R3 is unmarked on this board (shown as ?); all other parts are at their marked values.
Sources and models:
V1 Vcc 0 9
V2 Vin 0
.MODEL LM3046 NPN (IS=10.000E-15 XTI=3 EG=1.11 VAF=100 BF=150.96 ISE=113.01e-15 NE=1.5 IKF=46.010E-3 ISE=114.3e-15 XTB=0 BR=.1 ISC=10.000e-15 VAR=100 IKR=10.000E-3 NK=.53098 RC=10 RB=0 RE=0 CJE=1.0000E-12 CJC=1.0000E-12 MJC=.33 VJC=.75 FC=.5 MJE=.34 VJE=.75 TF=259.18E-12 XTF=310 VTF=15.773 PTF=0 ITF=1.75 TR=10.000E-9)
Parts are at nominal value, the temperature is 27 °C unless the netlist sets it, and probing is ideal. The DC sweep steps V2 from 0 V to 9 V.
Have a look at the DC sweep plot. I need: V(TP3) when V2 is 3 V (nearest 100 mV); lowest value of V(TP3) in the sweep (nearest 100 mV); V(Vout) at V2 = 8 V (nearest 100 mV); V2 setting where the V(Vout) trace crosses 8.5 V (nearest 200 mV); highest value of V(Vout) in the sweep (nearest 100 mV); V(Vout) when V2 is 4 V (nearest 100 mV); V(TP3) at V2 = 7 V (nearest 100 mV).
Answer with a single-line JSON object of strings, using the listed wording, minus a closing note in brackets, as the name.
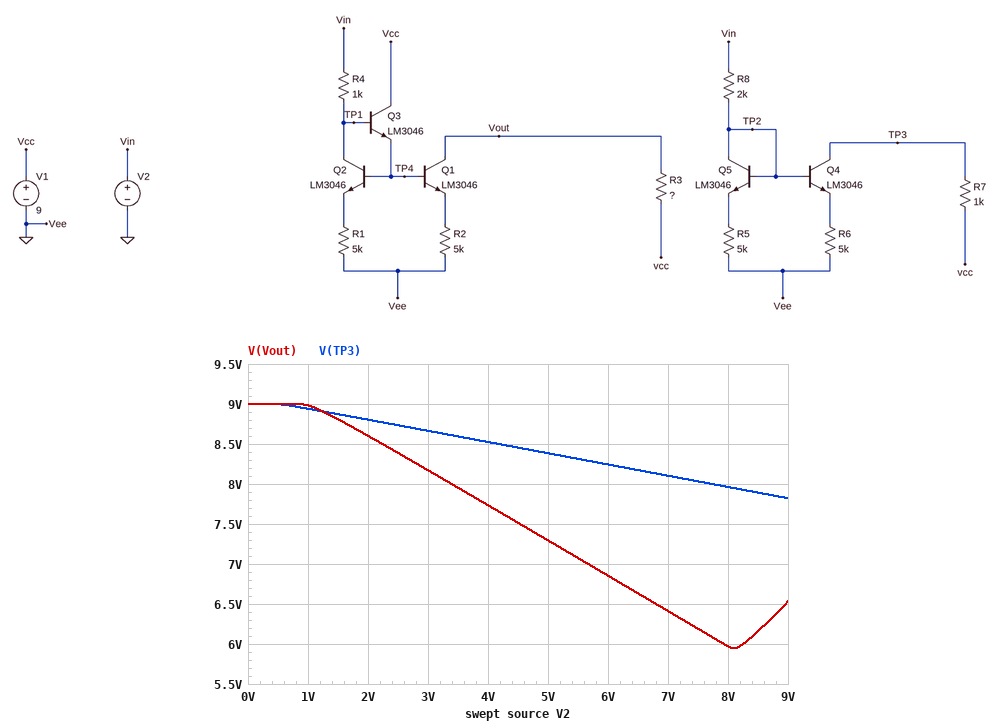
{"V(TP3) when V2 is 3 V": "8.7 V", "lowest value of V(TP3) in the sweep": "7.8 V", "V(Vout) at V2 = 8 V": "6.0 V", "V2 setting where the V(Vout) trace crosses 8.5 V": "2.2 V", "highest value of V(Vout) in the sweep": "9.0 V", "V(Vout) when V2 is 4 V": "7.7 V", "V(TP3) at V2 = 7 V": "8.1 V"}
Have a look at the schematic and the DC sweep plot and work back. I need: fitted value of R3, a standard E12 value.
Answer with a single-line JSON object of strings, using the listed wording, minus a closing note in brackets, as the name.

{"fitted value of R3, a standard E12 value": "2.7 kΩ"}
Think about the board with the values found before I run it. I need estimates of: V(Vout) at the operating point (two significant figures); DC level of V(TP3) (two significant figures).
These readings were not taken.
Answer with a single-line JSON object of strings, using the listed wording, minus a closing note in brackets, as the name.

{"V(Vout) at the operating point": "9.0 V", "DC level of V(TP3)": "9.0 V"}
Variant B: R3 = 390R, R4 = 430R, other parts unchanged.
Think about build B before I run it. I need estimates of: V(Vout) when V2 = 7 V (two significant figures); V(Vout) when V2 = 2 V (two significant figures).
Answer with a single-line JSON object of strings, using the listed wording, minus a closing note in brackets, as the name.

{"V(Vout) when V2 = 7 V": "8.6 V", "V(Vout) when V2 = 2 V": "8.9 V"}
